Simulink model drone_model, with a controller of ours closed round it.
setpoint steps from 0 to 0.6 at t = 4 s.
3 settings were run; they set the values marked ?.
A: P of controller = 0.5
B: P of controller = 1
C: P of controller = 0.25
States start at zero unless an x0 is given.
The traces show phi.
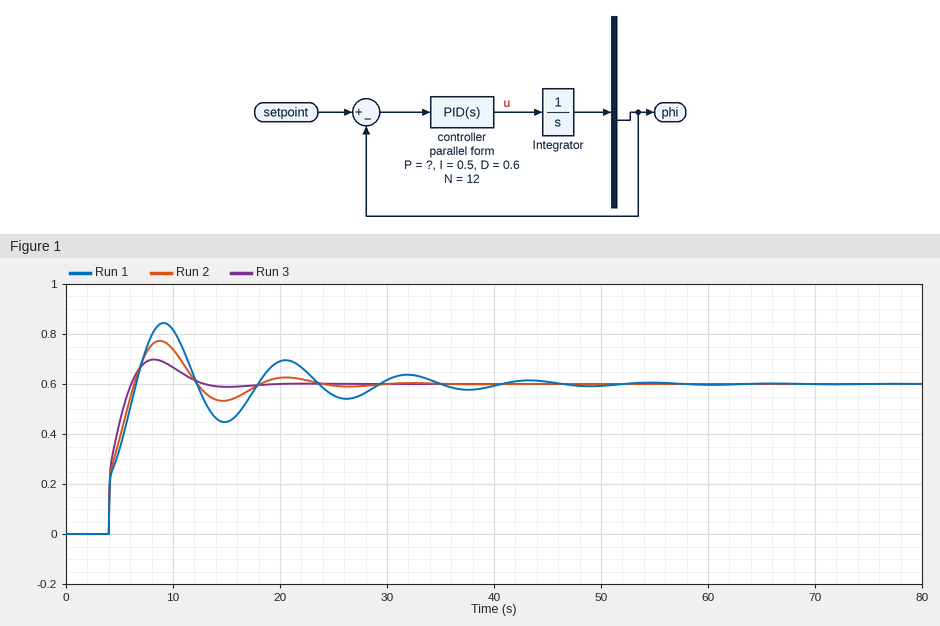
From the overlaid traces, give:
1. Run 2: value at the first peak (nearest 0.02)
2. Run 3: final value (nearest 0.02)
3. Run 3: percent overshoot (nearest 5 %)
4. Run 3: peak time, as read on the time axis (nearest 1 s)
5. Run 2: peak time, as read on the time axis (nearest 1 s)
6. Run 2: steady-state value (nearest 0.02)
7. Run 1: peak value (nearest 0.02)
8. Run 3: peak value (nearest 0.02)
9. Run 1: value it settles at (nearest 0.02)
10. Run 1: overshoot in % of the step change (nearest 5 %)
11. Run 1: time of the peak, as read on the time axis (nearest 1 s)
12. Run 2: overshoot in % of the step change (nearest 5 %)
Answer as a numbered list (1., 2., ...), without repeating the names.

1. 0.78
2. 0.60
3. 15 %
4. 8 s
5. 9 s
6. 0.60
7. 0.84
8. 0.70
9. 0.60
10. 40 %
11. 9 s
12. 30 %
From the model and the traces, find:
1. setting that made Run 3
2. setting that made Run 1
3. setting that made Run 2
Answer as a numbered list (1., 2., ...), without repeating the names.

1. B
2. C
3. A
